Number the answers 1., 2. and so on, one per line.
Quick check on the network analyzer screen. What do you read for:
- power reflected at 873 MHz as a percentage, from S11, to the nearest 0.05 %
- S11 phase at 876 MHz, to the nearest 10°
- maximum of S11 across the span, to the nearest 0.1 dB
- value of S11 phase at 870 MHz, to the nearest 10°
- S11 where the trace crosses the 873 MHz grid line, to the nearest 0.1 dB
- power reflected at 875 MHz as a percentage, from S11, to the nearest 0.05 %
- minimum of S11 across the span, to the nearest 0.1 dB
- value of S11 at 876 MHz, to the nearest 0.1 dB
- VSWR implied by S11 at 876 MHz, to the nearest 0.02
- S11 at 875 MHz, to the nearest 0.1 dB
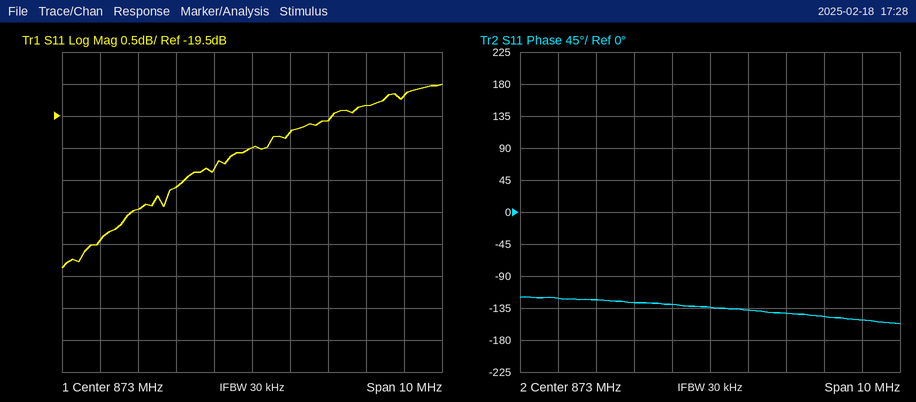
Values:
1. 1.00 %
2. -150°
3. -19.0 dB
4. -120°
5. -20.0 dB
6. 1.10 %
7. -21.9 dB
8. -19.3 dB
9. 1.24
10. -19.6 dB
